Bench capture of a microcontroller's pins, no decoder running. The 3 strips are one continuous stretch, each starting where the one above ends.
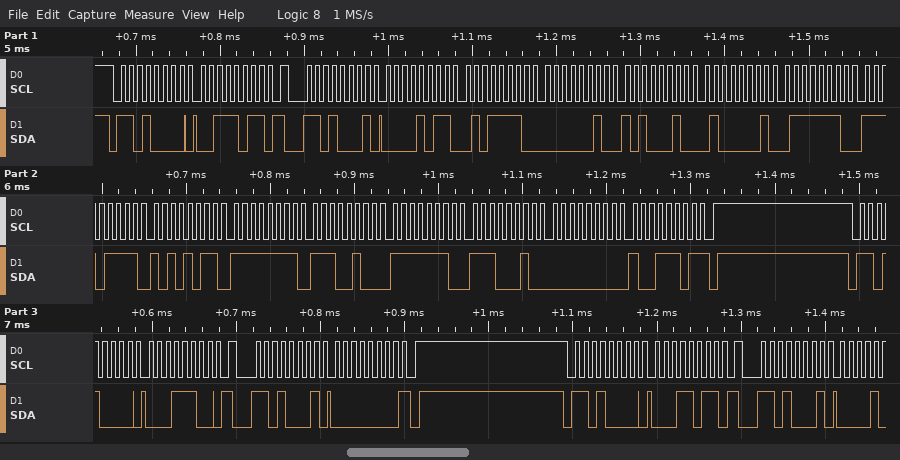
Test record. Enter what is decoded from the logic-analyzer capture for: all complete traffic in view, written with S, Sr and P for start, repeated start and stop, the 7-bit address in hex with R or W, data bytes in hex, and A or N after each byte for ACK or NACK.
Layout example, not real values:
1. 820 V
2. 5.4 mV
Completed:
1. S 68W A 3B A Sr 68R A 0B A 5E A 02 A A2 A 41 A 7E A EF A AB A FF A E4 A FE A E2 A 00 A 9D N P S 68W A 1C A Sr 68R A 00 N P S 68W A 1B A Sr 68R A
